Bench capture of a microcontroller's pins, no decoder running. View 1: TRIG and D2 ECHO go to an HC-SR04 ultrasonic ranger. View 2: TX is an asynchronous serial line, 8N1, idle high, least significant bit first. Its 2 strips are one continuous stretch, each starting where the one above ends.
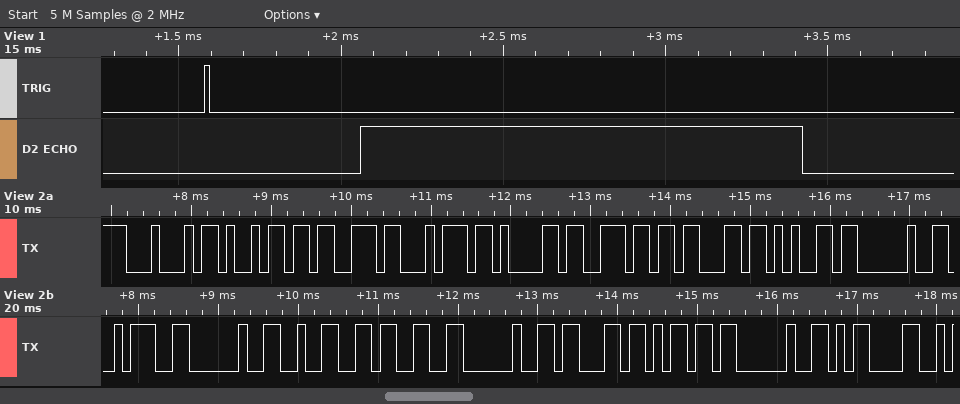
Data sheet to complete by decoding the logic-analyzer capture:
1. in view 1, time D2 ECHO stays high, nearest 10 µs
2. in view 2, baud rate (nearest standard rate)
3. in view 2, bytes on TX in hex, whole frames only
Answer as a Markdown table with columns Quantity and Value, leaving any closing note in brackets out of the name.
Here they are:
| Quantity | Value |
|---|---|
| in view 1, time D2 ECHO stays high, nearest 10 µs | 1360 µs |
| in view 2, baud rate | 9600 baud |
| in view 2, bytes on TX in hex, whole frames only | 0x44 0x69 0x73 0x74 0x61 0x6E 0x63 0x65 0x20 0x3A 0x20 0x32 0x33 0x20 0x63 0x6D 0x20 0x0D |
